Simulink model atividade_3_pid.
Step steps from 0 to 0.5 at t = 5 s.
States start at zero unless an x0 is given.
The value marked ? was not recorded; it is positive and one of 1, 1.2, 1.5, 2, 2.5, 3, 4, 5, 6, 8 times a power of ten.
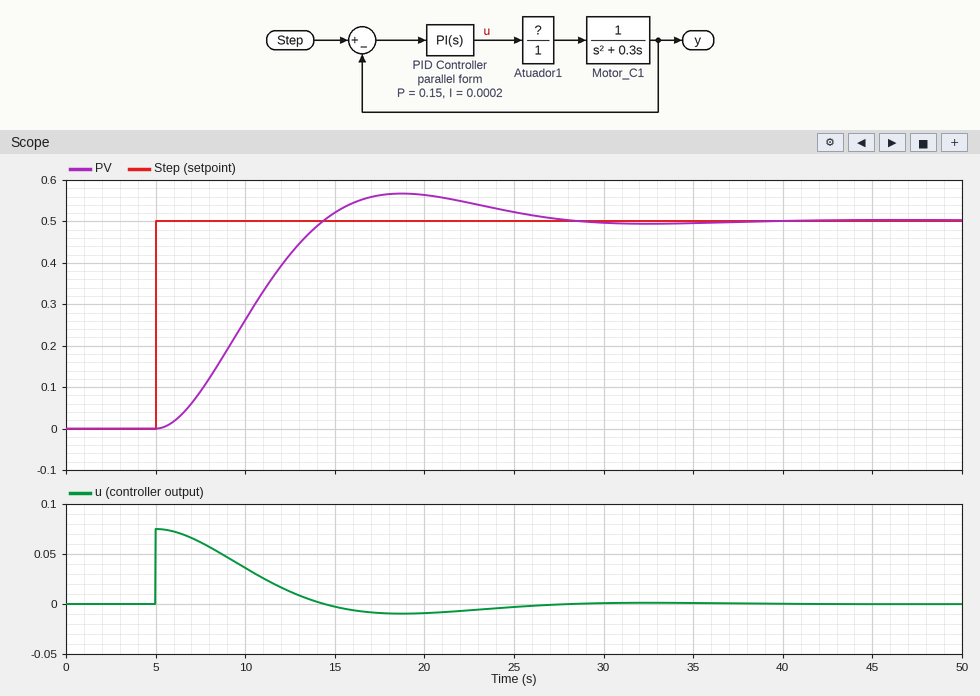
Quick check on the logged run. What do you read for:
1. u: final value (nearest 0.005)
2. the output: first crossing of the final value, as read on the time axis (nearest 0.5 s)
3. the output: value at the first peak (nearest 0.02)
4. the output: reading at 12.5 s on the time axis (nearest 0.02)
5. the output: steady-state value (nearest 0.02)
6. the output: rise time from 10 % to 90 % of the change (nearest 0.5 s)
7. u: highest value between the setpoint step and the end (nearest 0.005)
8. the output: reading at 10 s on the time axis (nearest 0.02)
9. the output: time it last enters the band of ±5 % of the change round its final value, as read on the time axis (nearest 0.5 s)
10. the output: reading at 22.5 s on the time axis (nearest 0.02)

0.000
14.5 s
0.56
0.42
0.50
6.5 s
0.075
0.26
24.5 s
0.54
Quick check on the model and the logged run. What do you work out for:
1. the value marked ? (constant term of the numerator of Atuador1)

0.5
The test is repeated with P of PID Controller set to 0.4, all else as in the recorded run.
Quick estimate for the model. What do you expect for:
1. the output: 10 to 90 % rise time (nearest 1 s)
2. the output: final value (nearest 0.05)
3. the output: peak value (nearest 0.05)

3 s
0.50
0.65
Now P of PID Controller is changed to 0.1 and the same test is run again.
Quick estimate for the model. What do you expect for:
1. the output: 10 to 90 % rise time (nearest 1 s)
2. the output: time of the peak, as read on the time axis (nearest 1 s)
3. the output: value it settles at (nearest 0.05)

9 s
24 s
0.50
